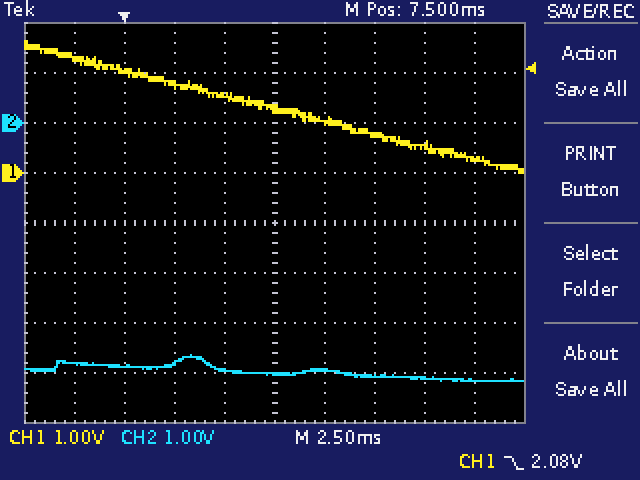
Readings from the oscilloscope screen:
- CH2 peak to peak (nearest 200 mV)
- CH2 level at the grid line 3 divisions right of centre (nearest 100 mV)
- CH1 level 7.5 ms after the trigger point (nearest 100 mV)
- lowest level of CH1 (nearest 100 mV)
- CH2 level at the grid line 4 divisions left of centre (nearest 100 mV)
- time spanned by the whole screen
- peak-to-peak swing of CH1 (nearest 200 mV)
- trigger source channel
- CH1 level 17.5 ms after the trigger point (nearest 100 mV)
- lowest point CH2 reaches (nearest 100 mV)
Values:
600 mV
-5.1 V
1.3 V
0.0 V
-4.8 V
25 ms
2.6 V
CH1
300 mV
-5.2 V
